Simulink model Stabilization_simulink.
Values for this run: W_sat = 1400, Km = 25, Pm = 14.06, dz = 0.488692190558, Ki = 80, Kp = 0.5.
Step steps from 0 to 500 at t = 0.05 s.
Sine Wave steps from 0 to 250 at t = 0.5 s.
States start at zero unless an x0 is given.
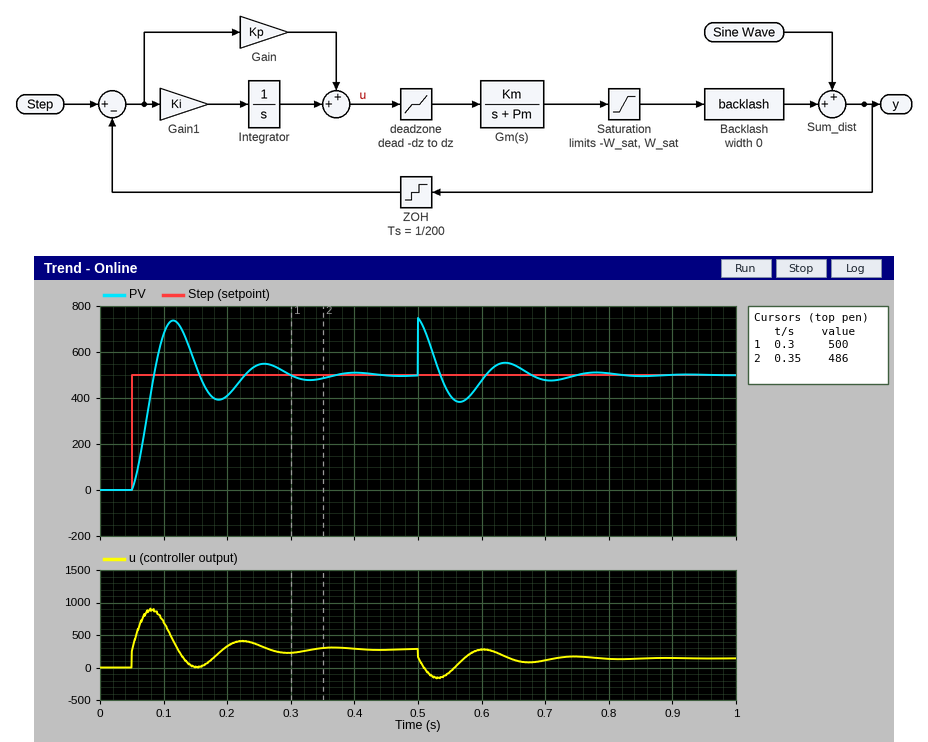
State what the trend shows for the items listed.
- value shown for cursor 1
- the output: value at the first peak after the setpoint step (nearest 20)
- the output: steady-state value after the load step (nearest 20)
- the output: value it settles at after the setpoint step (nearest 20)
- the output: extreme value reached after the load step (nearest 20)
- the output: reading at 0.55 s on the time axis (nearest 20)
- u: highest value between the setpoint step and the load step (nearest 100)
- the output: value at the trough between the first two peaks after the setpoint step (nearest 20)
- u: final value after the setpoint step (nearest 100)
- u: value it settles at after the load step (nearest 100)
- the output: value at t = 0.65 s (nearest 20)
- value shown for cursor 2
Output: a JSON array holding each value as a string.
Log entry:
["500", "740", "500", "500", "740", "420", "900", "400", "300", "100", "540", "486"]
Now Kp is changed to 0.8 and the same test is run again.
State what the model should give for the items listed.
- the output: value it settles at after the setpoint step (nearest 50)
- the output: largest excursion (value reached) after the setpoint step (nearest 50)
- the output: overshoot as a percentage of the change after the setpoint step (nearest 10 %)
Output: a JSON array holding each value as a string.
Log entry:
["500", "700", "40 %"]
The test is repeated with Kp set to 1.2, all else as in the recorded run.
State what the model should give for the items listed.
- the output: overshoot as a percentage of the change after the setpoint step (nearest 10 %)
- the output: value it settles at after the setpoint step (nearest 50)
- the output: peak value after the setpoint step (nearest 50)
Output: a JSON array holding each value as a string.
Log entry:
["30 %", "500", "650"]
